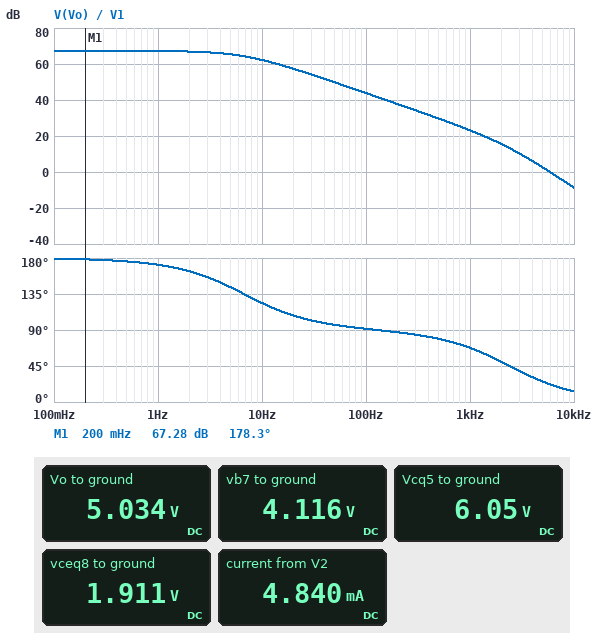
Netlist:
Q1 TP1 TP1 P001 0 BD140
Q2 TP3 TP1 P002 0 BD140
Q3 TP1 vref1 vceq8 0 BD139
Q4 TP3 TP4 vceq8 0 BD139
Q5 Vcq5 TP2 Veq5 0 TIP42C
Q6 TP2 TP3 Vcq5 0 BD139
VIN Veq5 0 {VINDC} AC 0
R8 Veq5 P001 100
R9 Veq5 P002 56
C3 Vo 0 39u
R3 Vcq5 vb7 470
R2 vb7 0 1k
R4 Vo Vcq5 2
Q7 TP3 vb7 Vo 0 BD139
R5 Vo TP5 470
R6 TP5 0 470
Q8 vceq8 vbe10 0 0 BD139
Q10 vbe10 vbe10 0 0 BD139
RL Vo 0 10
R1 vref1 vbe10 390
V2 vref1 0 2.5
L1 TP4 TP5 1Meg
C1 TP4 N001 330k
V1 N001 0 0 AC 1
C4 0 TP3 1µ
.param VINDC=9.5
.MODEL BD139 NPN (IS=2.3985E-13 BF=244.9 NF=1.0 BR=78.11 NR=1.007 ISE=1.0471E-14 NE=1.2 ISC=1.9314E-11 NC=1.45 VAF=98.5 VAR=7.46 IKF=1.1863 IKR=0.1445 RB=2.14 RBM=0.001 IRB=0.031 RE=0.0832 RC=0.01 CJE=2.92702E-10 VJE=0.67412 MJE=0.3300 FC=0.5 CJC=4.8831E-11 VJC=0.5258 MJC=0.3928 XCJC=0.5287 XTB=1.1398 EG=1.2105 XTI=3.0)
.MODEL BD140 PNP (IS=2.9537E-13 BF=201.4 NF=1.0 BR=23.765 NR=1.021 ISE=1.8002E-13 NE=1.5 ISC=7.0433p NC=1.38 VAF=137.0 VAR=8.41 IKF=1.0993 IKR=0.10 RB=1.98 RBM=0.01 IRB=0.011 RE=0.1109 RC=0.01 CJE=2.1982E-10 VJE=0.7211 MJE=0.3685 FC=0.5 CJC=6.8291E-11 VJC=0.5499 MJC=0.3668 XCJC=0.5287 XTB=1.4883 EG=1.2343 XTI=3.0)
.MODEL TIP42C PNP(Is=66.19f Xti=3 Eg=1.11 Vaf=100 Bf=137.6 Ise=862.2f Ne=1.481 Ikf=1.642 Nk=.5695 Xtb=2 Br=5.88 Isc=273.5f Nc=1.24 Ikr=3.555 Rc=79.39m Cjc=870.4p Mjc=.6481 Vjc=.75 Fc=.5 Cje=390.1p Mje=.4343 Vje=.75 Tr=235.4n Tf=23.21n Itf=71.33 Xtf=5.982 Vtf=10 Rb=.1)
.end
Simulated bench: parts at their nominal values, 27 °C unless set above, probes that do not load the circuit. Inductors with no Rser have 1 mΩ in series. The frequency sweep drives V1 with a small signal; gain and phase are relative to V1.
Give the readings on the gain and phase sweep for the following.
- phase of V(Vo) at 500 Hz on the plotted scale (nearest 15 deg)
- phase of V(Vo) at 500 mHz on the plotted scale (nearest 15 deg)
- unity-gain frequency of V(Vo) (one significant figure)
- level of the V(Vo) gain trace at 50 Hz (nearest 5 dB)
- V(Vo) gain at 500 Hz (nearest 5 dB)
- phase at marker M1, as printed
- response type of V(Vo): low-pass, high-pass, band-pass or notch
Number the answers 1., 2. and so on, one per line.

1. 75 deg
2. 180 deg
3. 6 kHz
4. 50 dB
5. 30 dB
6. 178.3 deg
7. low-pass
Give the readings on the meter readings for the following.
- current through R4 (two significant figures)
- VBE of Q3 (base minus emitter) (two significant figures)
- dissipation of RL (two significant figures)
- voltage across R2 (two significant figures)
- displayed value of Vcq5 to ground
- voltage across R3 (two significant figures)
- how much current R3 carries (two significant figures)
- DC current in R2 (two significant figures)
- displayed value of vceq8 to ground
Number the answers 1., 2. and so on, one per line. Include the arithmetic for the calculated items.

1. (6.05 V - 5.034 V) / 2 Ω = 510 mA
2. 2.5 V - 1.911 V = 590 mV
3. (5.034 V)^2 / 10 Ω = 2.5 W
4. 4.116 V = 4.1 V
5. 6.05 V
6. 6.05 V - 4.116 V = 1.9 V
7. (6.05 V - 4.116 V) / 470 Ω = 4.1 mA
8. (4.116 V) / 1 kΩ = 4.1 mA
9. 1.911 V
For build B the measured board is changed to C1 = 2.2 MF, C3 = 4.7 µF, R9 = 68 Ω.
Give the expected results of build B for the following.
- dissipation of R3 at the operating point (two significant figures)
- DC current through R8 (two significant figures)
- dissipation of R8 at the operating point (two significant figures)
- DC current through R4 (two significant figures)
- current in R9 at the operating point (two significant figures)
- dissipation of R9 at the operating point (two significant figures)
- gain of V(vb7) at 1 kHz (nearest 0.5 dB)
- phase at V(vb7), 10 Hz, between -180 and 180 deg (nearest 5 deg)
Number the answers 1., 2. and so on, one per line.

1. 7.9 mW
2. 2.0 mA
3. 410 µW
4. 510 mA
5. 2.8 mA
6. 550 µW
7. 21.5 dB
8. 120 deg
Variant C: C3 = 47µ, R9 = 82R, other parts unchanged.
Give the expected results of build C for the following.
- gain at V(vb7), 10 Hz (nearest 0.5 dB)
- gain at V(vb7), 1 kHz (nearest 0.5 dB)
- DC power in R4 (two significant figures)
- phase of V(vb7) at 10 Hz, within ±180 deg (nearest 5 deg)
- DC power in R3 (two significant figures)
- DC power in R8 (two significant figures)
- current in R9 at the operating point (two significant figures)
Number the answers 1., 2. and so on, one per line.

1. 59.5 dB
2. 20.5 dB
3. 510 mW
4. 120 deg
5. 7.9 mW
6. 490 µW
7. 2.6 mA
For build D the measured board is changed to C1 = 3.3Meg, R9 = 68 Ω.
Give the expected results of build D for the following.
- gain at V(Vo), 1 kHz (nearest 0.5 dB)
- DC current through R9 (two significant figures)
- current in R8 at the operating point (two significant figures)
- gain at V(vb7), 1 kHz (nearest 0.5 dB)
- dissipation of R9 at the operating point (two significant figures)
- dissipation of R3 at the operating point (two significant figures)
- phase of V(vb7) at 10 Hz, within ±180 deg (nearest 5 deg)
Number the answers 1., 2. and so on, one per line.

1. 22.5 dB
2. 2.8 mA
3. 2.0 mA
4. 21.5 dB
5. 550 µW
6. 7.9 mW
7. 120 deg
